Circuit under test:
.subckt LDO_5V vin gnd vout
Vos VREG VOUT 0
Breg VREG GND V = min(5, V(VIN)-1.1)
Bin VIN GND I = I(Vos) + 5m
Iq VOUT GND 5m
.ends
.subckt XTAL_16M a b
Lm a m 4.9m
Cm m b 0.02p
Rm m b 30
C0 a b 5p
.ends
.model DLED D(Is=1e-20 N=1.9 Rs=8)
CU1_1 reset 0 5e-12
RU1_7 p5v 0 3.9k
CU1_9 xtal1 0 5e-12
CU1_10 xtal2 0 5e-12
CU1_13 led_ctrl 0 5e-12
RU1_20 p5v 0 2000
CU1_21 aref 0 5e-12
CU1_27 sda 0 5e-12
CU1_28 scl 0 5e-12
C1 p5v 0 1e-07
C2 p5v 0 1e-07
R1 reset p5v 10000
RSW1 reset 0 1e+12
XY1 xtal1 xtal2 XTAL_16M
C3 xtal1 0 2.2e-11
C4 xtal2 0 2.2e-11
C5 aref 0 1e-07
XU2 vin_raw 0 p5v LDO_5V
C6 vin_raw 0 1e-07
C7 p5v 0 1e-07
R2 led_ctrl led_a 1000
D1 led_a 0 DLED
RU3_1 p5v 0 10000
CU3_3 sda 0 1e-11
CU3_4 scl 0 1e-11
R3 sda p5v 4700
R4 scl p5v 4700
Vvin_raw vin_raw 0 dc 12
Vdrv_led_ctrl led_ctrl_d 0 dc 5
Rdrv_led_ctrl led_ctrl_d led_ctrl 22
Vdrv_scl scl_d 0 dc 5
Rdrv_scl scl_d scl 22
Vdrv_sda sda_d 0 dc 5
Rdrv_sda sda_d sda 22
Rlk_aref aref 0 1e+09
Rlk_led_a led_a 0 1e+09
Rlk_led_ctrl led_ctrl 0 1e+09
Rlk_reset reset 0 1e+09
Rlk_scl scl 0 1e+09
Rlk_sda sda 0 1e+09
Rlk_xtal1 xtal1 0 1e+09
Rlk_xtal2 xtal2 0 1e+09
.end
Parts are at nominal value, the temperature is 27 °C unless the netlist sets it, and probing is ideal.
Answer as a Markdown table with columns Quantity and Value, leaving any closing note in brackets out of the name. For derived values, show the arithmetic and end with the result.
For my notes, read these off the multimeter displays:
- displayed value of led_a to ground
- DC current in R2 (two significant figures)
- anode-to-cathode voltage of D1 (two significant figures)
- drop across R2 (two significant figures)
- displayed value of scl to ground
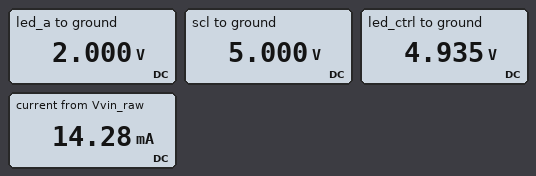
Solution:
| Quantity | Value |
|---|---|
| displayed value of led_a to ground | 2.000 V |
| DC current in R2 | (4.935 V - 2 V) / 1 kΩ = 2.9 mA |
| anode-to-cathode voltage of D1 | 2 V = 2.0 V |
| drop across R2 | 4.935 V - 2 V = 2.9 V |
| displayed value of scl to ground | 5.000 V |
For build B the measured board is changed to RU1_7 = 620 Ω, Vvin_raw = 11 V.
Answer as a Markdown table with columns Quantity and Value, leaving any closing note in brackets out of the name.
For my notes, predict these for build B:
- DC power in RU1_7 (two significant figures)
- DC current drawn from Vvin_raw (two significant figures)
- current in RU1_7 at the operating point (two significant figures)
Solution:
| Quantity | Value |
|---|---|
| DC power in RU1_7 | 40 mW |
| DC current drawn from Vvin_raw | 21 mA |
| current in RU1_7 at the operating point | 8.1 mA |
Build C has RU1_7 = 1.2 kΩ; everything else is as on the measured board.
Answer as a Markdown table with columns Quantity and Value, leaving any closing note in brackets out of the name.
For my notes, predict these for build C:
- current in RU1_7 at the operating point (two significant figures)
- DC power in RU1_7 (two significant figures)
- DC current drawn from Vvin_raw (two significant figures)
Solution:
| Quantity | Value |
|---|---|
| current in RU1_7 at the operating point | 4.2 mA |
| DC power in RU1_7 | 21 mW |
| DC current drawn from Vvin_raw | 17 mA |
